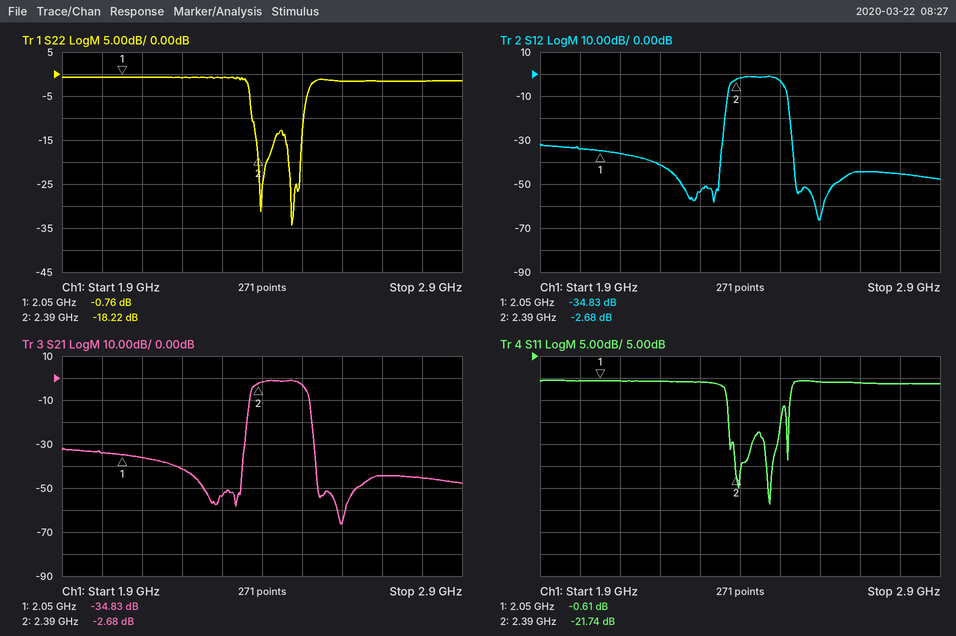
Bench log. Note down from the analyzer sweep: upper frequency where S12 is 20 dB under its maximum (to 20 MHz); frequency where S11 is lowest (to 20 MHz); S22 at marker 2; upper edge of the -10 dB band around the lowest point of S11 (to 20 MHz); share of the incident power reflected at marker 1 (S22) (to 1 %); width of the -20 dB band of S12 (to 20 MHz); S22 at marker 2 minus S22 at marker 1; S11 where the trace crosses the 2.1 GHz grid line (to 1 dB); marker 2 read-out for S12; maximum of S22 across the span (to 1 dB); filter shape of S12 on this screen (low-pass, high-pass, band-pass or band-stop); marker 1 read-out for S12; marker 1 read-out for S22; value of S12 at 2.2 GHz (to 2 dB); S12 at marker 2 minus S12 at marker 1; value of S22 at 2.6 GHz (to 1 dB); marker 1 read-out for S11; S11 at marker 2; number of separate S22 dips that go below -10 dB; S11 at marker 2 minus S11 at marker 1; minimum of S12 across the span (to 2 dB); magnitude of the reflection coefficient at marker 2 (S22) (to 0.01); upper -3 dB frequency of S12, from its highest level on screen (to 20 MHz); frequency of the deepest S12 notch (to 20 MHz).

2.52 GHz
2.48 GHz
-18.22 dB
2.50 GHz
84 %
160 MHz
-17.46 dB
-1 dB
-2.68 dB
-1 dB
band-pass
-34.83 dB
-0.76 dB
-42 dB
32.15 dB
-2 dB
-0.61 dB
-21.74 dB
2
-21.13 dB
-66 dB
0.12
2.50 GHz
2.60 GHz
